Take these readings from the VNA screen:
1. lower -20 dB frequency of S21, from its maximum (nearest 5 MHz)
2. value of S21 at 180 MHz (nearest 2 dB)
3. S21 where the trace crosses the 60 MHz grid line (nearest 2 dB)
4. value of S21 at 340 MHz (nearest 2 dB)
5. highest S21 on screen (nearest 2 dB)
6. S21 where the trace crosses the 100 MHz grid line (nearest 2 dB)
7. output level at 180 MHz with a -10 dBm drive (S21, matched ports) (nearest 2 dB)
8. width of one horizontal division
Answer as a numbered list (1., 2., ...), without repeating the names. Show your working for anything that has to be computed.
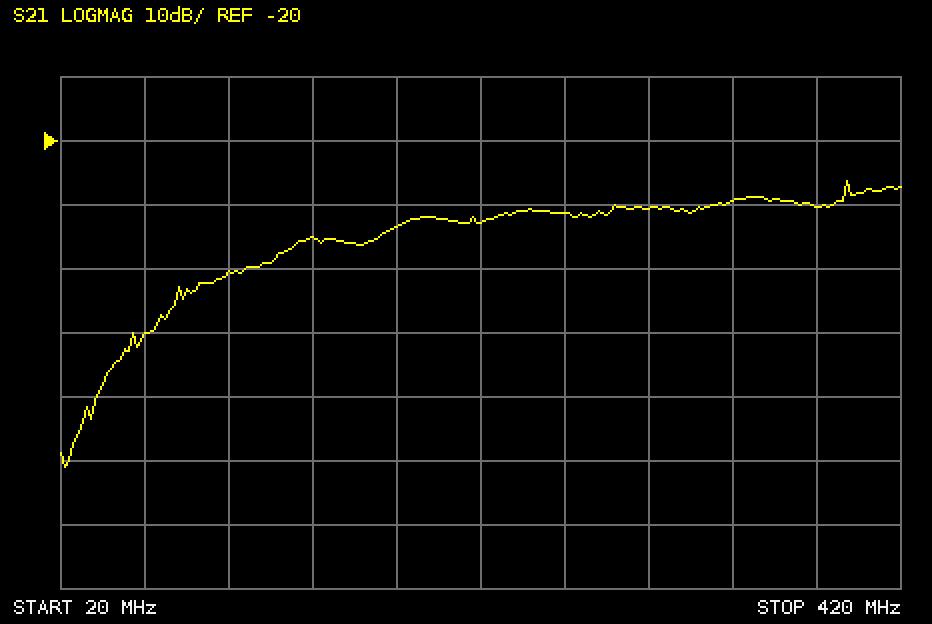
1. 70 MHz
2. -34 dB
3. -50 dB
4. -30 dB
5. -26 dB
6. -40 dB
7. -10 dBm + (-34 dB) = -44 dBm
8. 40 MHz
